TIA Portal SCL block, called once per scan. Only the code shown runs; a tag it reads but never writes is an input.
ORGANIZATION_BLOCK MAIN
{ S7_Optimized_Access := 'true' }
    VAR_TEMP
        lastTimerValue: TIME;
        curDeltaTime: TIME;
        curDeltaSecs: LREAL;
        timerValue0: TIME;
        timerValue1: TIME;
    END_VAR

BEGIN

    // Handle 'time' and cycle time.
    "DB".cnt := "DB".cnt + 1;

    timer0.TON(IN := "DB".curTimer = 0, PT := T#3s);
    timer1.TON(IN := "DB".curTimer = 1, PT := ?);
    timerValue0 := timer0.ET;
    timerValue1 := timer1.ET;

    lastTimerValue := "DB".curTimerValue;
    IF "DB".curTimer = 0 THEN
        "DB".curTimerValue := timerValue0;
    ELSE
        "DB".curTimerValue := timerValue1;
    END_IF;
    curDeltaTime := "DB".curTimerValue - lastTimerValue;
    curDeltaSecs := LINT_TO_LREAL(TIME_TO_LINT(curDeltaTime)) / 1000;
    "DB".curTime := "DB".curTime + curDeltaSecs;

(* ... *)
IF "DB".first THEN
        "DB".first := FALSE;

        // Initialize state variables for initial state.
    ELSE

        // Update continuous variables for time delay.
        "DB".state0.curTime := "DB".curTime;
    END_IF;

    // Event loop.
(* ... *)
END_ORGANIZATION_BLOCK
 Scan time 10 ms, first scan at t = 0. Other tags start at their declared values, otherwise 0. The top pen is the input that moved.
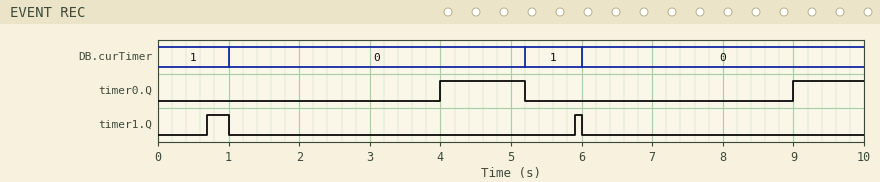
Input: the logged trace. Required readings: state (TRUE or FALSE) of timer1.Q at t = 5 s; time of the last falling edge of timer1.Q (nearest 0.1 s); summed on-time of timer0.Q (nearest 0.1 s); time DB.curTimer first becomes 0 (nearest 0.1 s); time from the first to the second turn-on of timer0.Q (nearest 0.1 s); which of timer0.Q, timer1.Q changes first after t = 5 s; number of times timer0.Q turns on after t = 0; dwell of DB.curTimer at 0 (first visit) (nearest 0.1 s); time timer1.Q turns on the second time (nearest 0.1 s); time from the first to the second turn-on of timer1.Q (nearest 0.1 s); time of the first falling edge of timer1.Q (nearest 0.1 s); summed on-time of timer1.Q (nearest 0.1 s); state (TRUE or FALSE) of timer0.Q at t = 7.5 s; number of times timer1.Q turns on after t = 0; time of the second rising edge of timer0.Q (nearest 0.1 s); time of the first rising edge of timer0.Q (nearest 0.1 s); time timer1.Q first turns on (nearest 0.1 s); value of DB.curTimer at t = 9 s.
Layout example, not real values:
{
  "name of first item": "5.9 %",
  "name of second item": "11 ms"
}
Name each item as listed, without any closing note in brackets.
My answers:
{
  "state (TRUE or FALSE) of timer1.Q at t = 5 s": "FALSE",
  "time of the last falling edge of timer1.Q": "6.0 s",
  "summed on-time of timer0.Q": "2.2 s",
  "time DB.curTimer first becomes 0": "1.0 s",
  "time from the first to the second turn-on of timer0.Q": "5.0 s",
  "which of timer0.Q, timer1.Q changes first after t = 5 s": "timer0.Q",
  "number of times timer0.Q turns on after t = 0": "2",
  "dwell of DB.curTimer at 0 (first visit)": "4.2 s",
  "time timer1.Q turns on the second time": "5.9 s",
  "time from the first to the second turn-on of timer1.Q": "5.2 s",
  "time of the first falling edge of timer1.Q": "1.0 s",
  "summed on-time of timer1.Q": "0.4 s",
  "state (TRUE or FALSE) of timer0.Q at t = 7.5 s": "FALSE",
  "number of times timer1.Q turns on after t = 0": "2",
  "time of the second rising edge of timer0.Q": "9.0 s",
  "time of the first rising edge of timer0.Q": "4.0 s",
  "time timer1.Q first turns on": "0.7 s",
  "value of DB.curTimer at t = 9 s": "0"
}
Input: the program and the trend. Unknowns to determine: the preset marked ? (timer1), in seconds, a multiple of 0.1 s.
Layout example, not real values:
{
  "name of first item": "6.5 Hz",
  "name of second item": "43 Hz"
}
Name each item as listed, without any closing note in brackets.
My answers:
{
  "the preset marked ? (timer1), in seconds, a multiple of 0.1 s": "0.7 s"
}
